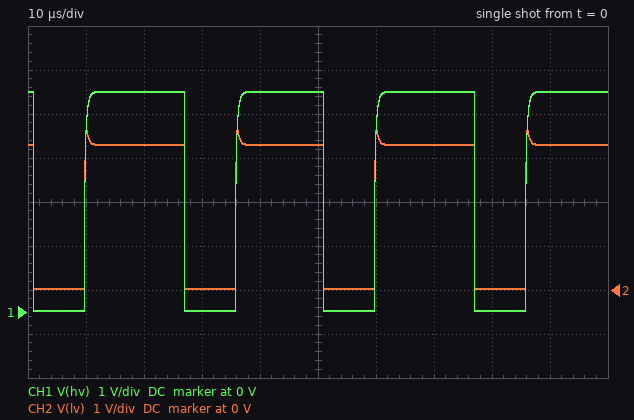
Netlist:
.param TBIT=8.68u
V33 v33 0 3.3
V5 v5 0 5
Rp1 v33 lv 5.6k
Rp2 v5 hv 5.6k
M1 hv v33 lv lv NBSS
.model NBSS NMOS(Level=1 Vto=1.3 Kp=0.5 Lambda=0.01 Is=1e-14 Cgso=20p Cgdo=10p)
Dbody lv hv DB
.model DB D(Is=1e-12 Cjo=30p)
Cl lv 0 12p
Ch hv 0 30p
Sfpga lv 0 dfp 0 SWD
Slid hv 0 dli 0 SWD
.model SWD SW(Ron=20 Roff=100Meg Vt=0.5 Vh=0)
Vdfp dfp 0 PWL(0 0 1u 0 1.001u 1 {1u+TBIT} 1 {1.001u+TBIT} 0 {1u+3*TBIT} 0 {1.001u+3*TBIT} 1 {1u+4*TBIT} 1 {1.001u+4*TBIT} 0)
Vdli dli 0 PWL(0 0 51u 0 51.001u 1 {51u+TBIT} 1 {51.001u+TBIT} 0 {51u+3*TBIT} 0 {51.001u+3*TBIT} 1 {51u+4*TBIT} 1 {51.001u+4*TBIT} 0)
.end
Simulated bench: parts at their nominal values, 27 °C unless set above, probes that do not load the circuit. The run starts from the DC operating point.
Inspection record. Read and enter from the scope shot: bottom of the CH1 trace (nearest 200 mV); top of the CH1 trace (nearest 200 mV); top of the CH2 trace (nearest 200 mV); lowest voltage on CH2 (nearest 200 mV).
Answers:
0 V
5.0 V
3.6 V
0 V
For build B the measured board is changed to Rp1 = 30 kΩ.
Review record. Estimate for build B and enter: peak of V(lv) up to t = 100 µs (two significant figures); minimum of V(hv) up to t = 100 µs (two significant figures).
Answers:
3.8 V
20 mV
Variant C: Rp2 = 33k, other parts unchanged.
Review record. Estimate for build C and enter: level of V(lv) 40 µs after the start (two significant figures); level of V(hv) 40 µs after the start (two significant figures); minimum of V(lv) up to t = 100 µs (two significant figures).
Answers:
3.3 V
4.8 V
15 mV
